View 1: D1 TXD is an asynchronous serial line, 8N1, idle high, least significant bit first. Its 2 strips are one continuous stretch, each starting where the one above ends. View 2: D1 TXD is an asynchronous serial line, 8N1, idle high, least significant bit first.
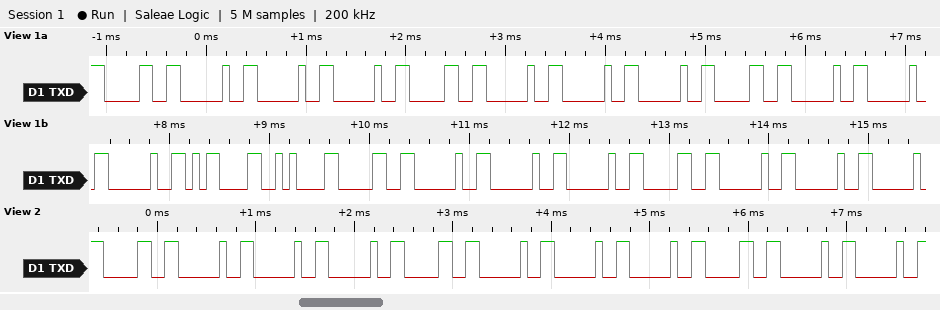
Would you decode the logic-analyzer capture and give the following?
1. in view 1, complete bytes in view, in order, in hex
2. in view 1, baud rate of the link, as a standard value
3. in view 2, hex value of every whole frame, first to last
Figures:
30 20 20 20 30 20 20 20 30 20 20 20 0D 0A 30 20 20 20 30 20 20
14400 baud
30 20 20 20 30 20 20 20 30 20 20
